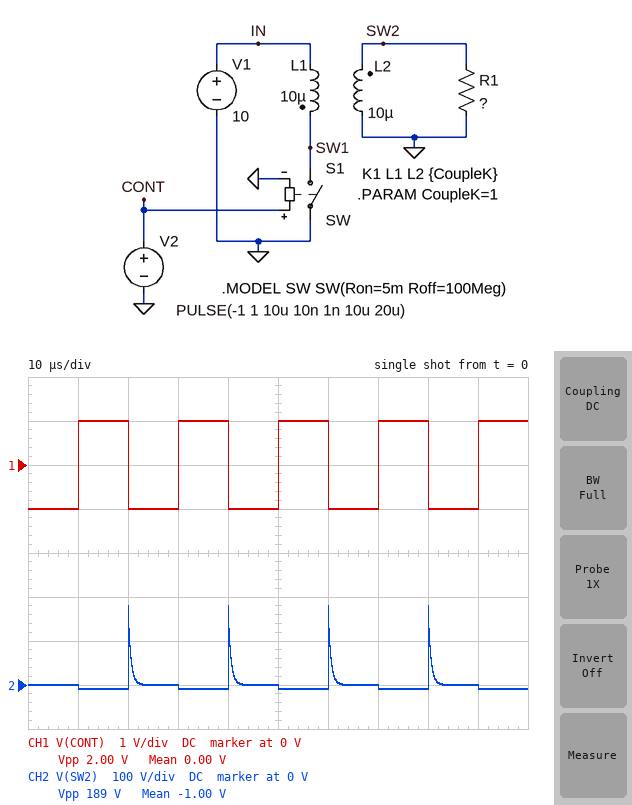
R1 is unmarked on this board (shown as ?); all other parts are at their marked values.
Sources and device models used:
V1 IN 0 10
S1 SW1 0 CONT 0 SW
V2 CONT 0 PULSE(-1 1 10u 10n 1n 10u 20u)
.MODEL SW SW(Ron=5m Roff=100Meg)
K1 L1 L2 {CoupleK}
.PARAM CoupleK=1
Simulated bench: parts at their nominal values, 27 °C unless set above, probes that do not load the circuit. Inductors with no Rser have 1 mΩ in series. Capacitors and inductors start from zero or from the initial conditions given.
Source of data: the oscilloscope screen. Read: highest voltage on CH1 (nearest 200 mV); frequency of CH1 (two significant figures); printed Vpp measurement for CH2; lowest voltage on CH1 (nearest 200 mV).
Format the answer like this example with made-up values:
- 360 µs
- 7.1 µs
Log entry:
- 1.0 V
- 50 kHz
- 189 V
- -1.0 V
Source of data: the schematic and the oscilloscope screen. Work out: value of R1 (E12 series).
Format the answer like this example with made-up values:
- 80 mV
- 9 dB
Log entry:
- 18 Ω
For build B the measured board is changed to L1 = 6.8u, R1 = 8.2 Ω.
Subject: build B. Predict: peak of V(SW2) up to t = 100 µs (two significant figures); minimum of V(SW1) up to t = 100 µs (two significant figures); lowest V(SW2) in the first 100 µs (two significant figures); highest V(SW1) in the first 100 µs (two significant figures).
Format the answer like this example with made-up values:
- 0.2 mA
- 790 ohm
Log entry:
- 99 V
- 9.0 mV
- -12 V
- 92 V
